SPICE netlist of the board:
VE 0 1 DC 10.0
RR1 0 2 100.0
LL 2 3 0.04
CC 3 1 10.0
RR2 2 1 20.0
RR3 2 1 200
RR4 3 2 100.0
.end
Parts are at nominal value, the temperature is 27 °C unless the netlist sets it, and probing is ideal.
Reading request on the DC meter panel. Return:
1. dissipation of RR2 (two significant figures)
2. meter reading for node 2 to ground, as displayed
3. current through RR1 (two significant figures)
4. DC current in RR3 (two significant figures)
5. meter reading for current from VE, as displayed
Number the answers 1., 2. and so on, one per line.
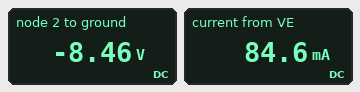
1. 120 mW
2. -8.46 V
3. 85 mA
4. 7.7 mA
5. 84.6 mA
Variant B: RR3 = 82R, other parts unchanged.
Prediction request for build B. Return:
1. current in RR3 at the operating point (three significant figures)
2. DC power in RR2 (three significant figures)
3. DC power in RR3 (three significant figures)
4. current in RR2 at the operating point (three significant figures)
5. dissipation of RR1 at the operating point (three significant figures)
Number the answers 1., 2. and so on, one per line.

1. 16.9 mA
2. 95.9 mW
3. 23.4 mW
4. 69.3 mA
5. 742 mW
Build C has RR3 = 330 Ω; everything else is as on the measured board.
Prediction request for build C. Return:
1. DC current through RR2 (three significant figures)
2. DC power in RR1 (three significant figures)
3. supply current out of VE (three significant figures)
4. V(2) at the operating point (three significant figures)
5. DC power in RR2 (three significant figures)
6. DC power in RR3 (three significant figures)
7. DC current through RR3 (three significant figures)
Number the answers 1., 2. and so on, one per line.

1. 79.3 mA
2. 708 mW
3. 84.1 mA
4. -8.41 V
5. 126 mW
6. 7.63 mW
7. 4.81 mA
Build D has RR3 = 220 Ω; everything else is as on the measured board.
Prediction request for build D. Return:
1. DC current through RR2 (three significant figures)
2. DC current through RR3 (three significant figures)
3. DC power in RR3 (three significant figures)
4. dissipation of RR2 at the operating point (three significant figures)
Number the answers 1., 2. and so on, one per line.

1. 77.5 mA
2. 7.04 mA
3. 10.9 mW
4. 120 mW
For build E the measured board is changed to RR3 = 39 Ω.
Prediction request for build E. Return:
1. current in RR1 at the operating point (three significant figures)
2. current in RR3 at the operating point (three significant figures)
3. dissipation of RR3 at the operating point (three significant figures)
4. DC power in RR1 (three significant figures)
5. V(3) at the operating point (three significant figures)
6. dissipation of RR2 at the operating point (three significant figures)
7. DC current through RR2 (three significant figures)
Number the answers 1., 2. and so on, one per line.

1. 88.3 mA
2. 29.9 mA
3. 35.0 mW
4. 780 mW
5. -8.83 V
6. 68.2 mW
7. 58.4 mA
